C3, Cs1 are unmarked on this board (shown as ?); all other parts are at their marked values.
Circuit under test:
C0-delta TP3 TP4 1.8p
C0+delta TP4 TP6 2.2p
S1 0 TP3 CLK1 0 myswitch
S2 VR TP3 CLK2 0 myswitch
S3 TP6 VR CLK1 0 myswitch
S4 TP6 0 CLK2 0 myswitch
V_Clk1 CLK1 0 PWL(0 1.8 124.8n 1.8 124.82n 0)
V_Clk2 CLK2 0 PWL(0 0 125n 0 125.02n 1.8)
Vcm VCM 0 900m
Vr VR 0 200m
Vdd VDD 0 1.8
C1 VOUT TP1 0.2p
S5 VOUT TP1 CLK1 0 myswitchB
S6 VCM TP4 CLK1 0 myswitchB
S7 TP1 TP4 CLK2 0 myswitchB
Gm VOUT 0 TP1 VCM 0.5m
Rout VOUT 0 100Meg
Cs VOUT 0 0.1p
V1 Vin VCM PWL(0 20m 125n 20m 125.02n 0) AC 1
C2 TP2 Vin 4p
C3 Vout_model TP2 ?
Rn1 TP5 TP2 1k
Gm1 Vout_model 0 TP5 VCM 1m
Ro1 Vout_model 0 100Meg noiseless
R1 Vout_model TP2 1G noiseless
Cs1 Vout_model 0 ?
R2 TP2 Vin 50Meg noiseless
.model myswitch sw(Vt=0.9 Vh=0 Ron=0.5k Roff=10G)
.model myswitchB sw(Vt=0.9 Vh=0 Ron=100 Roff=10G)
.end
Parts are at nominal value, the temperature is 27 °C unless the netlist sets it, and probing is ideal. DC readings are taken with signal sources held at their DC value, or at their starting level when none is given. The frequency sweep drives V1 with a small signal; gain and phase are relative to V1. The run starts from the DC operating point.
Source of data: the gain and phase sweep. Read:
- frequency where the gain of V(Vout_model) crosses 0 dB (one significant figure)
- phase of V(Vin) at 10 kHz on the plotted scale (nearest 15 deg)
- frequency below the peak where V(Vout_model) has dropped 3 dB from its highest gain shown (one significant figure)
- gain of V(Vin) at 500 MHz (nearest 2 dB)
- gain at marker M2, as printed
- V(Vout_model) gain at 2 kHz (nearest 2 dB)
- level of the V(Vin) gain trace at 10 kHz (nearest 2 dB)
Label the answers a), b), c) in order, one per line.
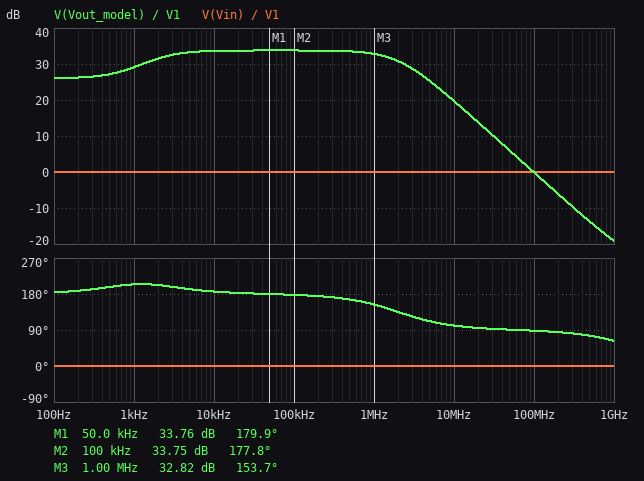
a) 100 MHz
b) 0 deg
c) 2 kHz
d) 0 dB
e) 33.75 dB
f) 32 dB
g) 0 dB
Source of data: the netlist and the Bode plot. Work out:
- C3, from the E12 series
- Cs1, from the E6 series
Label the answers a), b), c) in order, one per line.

a) 82 fF
b) 1.5 pF
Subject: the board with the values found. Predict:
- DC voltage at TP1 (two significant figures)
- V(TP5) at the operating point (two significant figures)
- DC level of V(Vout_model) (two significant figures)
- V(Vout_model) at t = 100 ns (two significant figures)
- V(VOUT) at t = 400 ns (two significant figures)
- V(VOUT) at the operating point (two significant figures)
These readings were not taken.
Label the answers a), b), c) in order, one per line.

a) 900 mV
b) 900 mV
c) 500 mV
d) 500 mV
e) 1.3 V
f) 900 mV
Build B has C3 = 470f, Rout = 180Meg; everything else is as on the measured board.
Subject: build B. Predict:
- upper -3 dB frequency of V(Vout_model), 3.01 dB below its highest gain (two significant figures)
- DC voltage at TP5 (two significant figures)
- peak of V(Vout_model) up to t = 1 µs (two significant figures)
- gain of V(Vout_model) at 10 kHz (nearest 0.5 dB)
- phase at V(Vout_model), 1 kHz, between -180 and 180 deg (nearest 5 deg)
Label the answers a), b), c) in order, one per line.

a) 420 Hz
b) 900 mV
c) 670 mV
d) 18.5 dB
e) 160 deg
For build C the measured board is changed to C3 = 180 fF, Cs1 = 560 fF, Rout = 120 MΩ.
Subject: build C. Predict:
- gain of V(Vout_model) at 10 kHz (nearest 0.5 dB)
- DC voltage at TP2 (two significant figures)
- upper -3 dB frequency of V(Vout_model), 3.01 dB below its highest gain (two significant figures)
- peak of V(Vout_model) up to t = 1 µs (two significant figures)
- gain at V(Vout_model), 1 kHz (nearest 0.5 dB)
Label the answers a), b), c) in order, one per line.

a) 27.0 dB
b) 900 mV
c) 9.4 MHz
d) 940 mV
e) 26.5 dB
